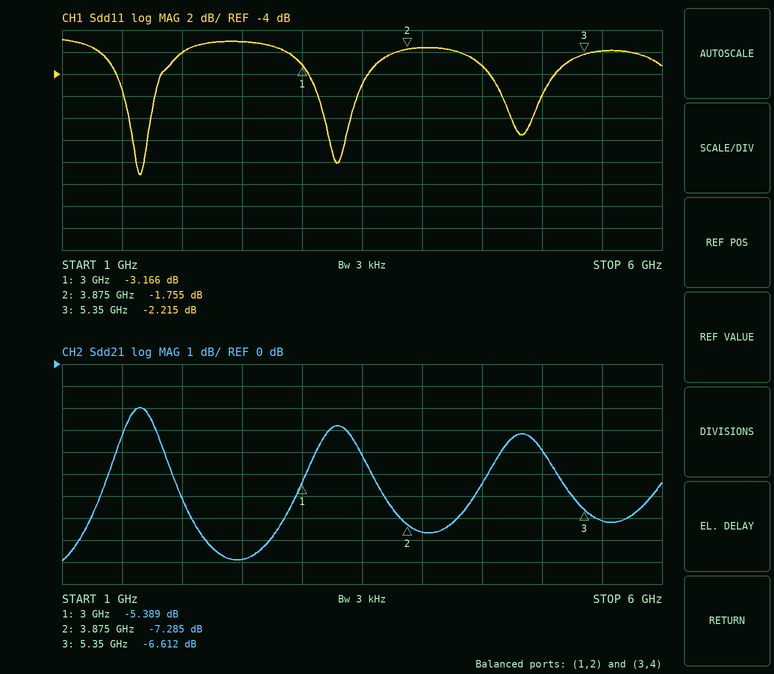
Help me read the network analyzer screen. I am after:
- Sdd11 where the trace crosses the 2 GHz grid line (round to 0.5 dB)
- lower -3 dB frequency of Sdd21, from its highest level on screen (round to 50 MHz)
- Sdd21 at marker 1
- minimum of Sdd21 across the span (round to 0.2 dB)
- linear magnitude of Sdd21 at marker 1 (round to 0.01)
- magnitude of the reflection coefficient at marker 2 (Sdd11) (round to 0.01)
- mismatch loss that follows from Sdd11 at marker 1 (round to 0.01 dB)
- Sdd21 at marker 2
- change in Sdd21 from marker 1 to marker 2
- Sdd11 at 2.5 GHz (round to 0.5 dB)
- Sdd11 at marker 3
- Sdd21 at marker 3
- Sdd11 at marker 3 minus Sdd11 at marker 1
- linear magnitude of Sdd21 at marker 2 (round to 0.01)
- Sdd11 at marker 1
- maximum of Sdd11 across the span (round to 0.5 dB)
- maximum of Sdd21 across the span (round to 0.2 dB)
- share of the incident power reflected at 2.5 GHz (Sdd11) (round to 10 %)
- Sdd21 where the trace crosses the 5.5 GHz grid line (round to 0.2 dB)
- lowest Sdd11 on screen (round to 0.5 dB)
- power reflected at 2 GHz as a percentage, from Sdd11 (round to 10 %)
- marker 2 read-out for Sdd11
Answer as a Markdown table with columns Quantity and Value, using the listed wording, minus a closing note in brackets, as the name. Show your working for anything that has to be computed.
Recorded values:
| Quantity | Value |
|---|---|
| Sdd11 where the trace crosses the 2 GHz grid line | -2.0 dB |
| lower -3 dB frequency of Sdd21, from its highest level on screen | 1.40 GHz |
| Sdd21 at marker 1 | -5.389 dB |
| minimum of Sdd21 across the span | -9.0 dB |
| linear magnitude of Sdd21 at marker 1 | 10^(-5.389/20) ≈ 0.54 |
| magnitude of the reflection coefficient at marker 2 (Sdd11) | 10^(-1.755/20) ≈ 0.82 |
| mismatch loss that follows from Sdd11 at marker 1 | −10 log10(1 − 10^(-3.166/10)) ≈ 2.86 dB |
| Sdd21 at marker 2 | -7.285 dB |
| change in Sdd21 from marker 1 to marker 2 | -7.285 − (-5.389) = -1.896 dB |
| Sdd11 at 2.5 GHz | -1.0 dB |
| Sdd11 at marker 3 | -2.215 dB |
| Sdd21 at marker 3 | -6.612 dB |
| Sdd11 at marker 3 minus Sdd11 at marker 1 | -2.215 − (-3.166) = 0.951 dB |
| linear magnitude of Sdd21 at marker 2 | 10^(-7.285/20) ≈ 0.43 |
| Sdd11 at marker 1 | -3.166 dB |
| maximum of Sdd11 across the span | -1.0 dB |
| maximum of Sdd21 across the span | -2.0 dB |
| share of the incident power reflected at 2.5 GHz (Sdd11) | 10^(-1/10) ≈ 79.4 %, so 80 % to the nearest 10 % |
| Sdd21 where the trace crosses the 5.5 GHz grid line | -7.2 dB |
| lowest Sdd11 on screen | -13.0 dB |
| power reflected at 2 GHz as a percentage, from Sdd11 | 10^(-2/10) ≈ 63.1 %, so 60 % to the nearest 10 % |
| marker 2 read-out for Sdd11 | -1.755 dB |
